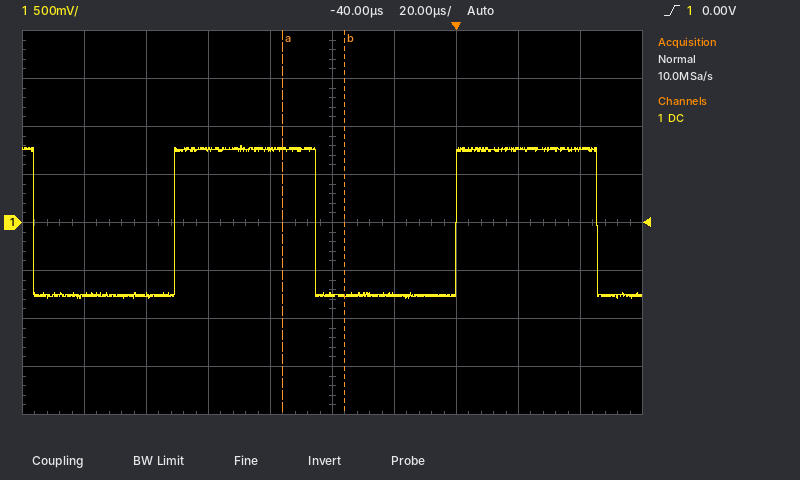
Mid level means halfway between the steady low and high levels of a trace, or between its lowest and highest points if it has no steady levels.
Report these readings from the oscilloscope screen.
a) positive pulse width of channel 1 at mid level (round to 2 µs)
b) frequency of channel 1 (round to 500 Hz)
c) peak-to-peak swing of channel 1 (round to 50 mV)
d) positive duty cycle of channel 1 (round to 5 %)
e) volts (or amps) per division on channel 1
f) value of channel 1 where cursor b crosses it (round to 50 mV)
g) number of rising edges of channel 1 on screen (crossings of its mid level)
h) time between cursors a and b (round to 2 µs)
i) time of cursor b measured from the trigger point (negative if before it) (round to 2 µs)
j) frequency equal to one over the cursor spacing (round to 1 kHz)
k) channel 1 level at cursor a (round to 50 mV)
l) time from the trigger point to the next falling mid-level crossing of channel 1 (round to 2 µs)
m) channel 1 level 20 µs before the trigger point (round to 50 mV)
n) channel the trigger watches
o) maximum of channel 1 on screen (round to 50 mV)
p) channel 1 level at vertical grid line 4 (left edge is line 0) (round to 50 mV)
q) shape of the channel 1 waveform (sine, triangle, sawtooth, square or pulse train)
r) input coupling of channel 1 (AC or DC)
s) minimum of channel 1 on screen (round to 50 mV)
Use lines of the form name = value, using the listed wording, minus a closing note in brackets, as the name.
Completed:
positive pulse width of channel 1 at mid level = 46 µs
frequency of channel 1 = 11.0 kHz
peak-to-peak swing of channel 1 = 1.60 V
positive duty cycle of channel 1 = 50 %
volts (or amps) per division on channel 1 = 500 mV
value of channel 1 where cursor b crosses it = -750 mV
number of rising edges of channel 1 on screen = 2
time between cursors a and b = 20 µs
time of cursor b measured from the trigger point (negative if before it) = -36 µs
frequency equal to one over the cursor spacing = 50 kHz
channel 1 level at cursor a = 750 mV
time from the trigger point to the next falling mid-level crossing of channel 1 = 46 µs
channel 1 level 20 µs before the trigger point = -750 mV
channel the trigger watches = channel 1
maximum of channel 1 on screen = 800 mV
channel 1 level at vertical grid line 4 (left edge is line 0) = 750 mV
shape of the channel 1 waveform = square
input coupling of channel 1 = DC
minimum of channel 1 on screen = -800 mV
